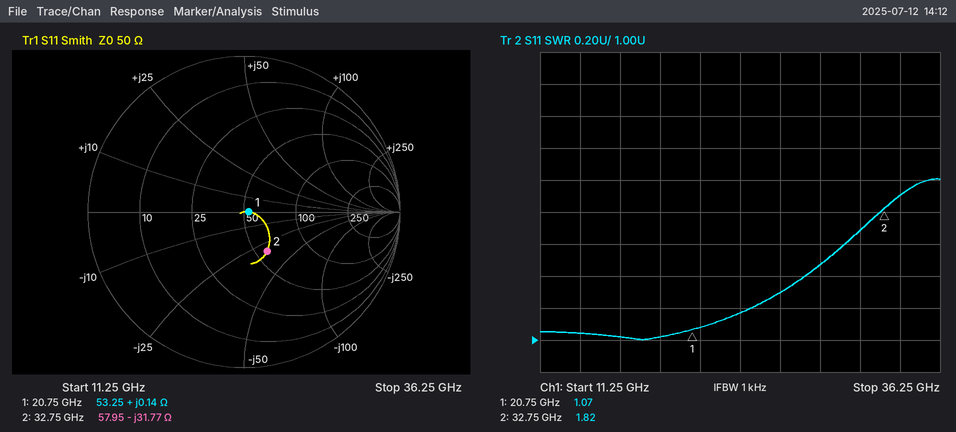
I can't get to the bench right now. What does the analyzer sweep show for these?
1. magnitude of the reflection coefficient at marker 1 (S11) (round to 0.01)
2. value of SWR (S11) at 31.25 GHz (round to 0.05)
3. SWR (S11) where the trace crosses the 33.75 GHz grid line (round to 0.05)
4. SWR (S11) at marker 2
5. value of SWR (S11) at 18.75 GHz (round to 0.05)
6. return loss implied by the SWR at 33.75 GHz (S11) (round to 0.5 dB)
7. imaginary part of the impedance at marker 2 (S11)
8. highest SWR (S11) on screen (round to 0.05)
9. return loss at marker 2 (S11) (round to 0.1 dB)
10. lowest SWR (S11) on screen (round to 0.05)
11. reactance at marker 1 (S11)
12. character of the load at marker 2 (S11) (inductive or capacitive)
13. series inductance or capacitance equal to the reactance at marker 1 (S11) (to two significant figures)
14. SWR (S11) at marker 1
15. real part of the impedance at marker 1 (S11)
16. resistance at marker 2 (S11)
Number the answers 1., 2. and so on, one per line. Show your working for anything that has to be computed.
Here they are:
1. 0.03
2. 1.70
3. 1.90
4. 1.82
5. 1.00
6. −20 log10((1.9 − 1)/(1.9 + 1)) ≈ 10.2 dB, so 10.0 dB to the nearest 0.5 dB
7. -31.77 Ω
8. 2.00
9. 10.7 dB
10. 1.00
11. +0.14 Ω
12. capacitive
13. L = 0.14 Ω/(2π × 20.75 GHz) ≈ 1.1 pH
14. 1.07
15. 53.25 Ω
16. 57.95 Ω
